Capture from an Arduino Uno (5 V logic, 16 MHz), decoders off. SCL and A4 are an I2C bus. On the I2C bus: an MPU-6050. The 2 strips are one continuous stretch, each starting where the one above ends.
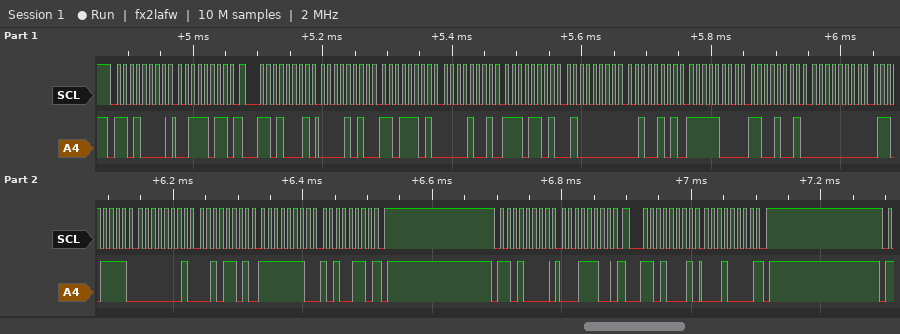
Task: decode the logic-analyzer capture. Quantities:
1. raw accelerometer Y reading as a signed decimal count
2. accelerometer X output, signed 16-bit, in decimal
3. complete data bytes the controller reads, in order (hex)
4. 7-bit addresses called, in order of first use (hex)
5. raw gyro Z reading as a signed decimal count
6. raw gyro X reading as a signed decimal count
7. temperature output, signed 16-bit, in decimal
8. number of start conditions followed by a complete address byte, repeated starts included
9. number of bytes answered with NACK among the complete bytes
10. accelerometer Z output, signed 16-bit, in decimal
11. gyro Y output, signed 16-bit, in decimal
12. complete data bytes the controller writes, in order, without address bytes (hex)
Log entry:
2541
2781
0A DD 09 ED 40 25 F8 C9 00 6F 01 2D FE A6 10
0x68
-346
111
-1847
4
2
16421
301
3B 1C
